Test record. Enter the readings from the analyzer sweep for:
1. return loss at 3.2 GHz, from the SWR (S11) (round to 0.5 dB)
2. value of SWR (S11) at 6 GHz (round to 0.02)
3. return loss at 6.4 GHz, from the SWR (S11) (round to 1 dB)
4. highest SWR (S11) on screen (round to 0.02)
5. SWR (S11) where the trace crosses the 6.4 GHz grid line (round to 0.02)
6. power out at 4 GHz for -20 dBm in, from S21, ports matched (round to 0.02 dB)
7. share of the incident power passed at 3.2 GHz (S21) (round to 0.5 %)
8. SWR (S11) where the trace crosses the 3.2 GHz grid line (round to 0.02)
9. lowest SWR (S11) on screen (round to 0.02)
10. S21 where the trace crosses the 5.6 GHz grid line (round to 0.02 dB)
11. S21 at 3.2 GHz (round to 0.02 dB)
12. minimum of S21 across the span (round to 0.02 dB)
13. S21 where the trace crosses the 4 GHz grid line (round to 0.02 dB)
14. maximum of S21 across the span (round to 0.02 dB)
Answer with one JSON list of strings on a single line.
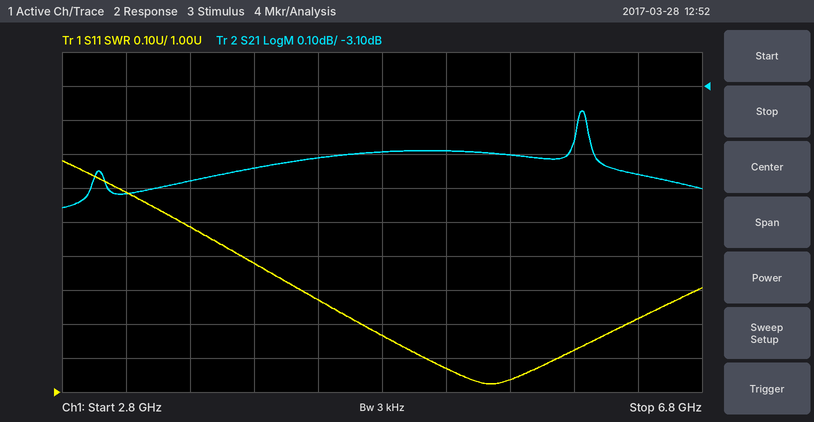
["13.0 dB", "1.12", "20 dB", "1.68", "1.22", "-23.34 dBm", "45.5 %", "1.58", "1.02", "-3.30 dB", "-3.42 dB", "-3.46 dB", "-3.34 dB", "-3.18 dB"]
